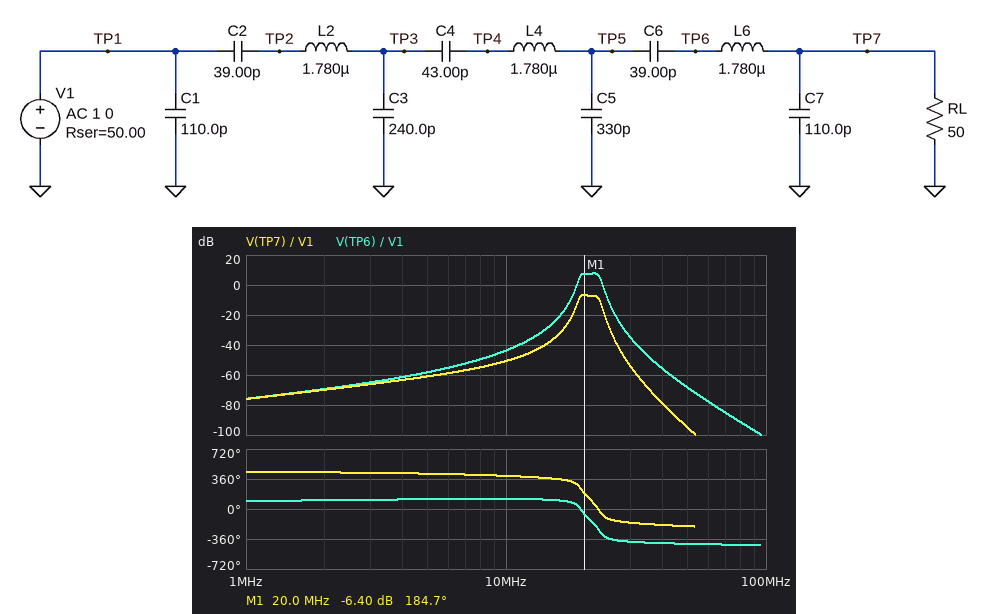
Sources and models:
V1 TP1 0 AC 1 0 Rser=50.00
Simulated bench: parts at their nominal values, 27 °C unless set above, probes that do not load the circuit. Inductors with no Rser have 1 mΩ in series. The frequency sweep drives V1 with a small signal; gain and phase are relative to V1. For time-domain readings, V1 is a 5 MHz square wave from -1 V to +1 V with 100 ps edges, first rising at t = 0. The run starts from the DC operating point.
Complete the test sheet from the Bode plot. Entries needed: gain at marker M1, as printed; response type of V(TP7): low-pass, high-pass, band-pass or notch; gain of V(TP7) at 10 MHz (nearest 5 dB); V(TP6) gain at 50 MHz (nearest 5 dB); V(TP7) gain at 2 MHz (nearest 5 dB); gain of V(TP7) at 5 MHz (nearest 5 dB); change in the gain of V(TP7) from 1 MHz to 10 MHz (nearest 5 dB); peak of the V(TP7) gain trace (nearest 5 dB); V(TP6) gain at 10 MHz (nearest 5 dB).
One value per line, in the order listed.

-6.40 dB
band-pass
-50 dB
-70 dB
-70 dB
-60 dB
25 dB
-5 dB
-45 dB
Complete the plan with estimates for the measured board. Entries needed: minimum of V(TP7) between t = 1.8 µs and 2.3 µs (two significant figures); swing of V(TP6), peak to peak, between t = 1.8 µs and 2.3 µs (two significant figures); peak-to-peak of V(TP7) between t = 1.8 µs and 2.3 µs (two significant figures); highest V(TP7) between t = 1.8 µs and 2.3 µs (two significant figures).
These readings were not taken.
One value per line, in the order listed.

-15 mV
170 mV
30 mV
15 mV
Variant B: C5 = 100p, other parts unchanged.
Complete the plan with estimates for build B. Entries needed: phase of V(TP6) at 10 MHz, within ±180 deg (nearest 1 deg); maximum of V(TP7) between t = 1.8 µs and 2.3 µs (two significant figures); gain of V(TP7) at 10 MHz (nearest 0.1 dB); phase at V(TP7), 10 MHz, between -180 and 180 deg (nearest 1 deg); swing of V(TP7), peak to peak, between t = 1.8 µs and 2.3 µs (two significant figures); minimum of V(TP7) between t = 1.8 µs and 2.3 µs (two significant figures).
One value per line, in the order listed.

123 deg
62 mV
-44.1 dB
39 deg
120 mV
-62 mV
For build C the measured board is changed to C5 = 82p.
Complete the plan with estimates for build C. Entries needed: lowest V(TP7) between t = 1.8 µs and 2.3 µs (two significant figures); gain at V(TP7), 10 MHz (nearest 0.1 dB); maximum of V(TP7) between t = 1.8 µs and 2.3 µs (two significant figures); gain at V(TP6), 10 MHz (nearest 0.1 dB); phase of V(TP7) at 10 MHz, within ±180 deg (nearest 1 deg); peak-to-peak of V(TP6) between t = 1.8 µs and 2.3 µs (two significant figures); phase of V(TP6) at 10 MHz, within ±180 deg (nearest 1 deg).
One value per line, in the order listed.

-47 mV
-43.3 dB
47 mV
-36.2 dB
39 deg
560 mV
123 deg
